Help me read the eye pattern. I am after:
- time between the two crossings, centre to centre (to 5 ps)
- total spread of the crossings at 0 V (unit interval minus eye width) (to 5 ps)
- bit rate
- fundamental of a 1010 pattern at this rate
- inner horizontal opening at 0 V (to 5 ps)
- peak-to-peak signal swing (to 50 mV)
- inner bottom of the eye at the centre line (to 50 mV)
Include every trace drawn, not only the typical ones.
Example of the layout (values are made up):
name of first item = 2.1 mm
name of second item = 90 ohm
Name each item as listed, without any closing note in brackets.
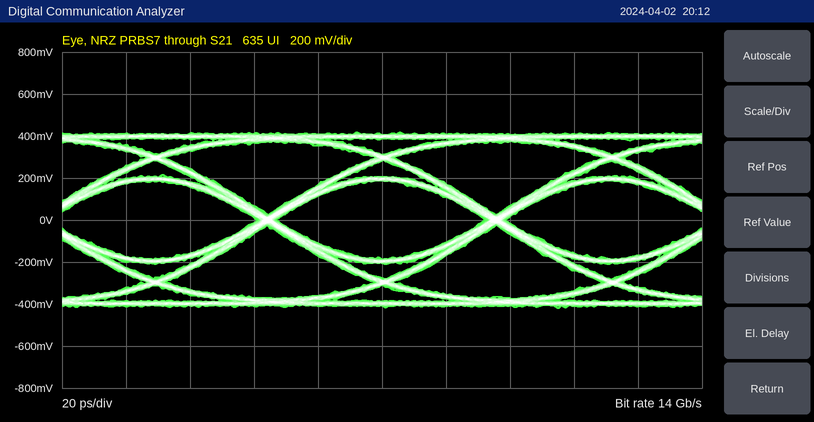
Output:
time between the two crossings, centre to centre = 70 ps
total spread of the crossings at 0 V (unit interval minus eye width) = 5 ps
bit rate = 14 Gb/s
fundamental of a 1010 pattern at this rate = 7 GHz
inner horizontal opening at 0 V = 65 ps
peak-to-peak signal swing = 850 mV
inner bottom of the eye at the centre line = -200 mV
